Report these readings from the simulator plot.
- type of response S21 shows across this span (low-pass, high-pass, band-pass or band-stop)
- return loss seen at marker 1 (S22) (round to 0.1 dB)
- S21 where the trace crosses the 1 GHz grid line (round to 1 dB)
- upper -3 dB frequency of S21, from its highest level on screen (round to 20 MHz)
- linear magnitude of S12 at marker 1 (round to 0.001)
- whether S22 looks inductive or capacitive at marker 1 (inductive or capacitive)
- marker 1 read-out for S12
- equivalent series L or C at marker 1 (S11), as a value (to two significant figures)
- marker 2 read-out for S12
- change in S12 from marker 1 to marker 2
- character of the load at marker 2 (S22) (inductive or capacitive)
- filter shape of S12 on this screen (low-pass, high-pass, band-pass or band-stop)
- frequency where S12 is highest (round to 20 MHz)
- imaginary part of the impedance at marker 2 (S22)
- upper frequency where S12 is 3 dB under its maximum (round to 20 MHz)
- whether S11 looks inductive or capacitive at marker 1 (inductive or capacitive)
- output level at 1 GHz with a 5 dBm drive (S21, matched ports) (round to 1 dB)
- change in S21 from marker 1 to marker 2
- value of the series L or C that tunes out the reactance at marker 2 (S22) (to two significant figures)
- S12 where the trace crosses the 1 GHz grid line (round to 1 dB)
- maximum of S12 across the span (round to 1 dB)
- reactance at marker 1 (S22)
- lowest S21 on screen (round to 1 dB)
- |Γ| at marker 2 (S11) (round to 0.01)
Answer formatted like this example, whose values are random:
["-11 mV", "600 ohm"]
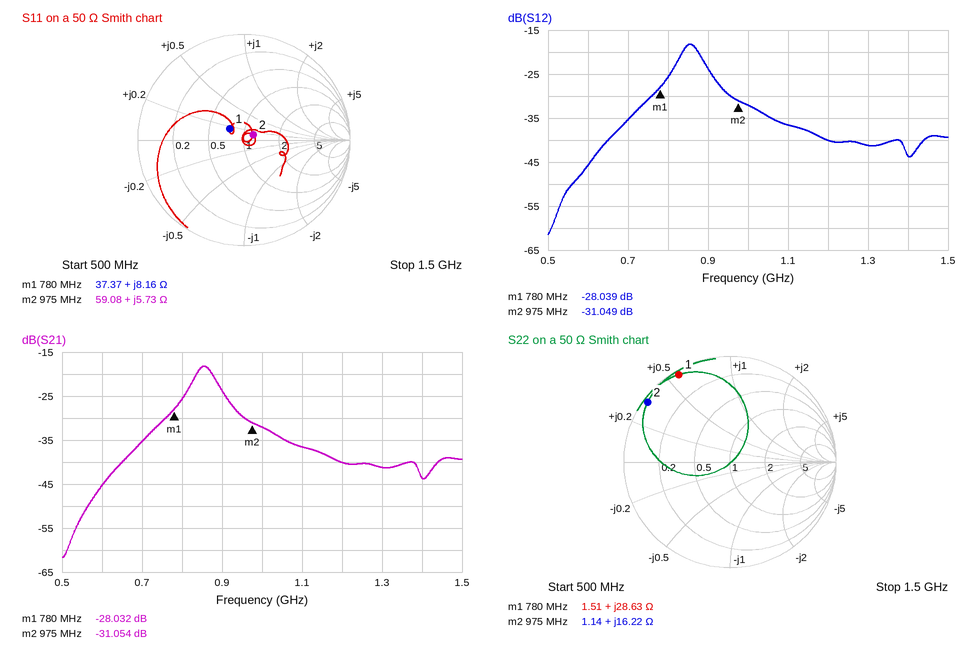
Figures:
["band-pass", "0.4 dB", "-32 dB", "880 MHz", "0.040", "inductive", "-28.039 dB", "1.7 nH", "-31.049 dB", "-3.010 dB", "inductive", "band-pass", "860 MHz", "+16.22 Ω", "880 MHz", "inductive", "-27 dBm", "-3.022 dB", "10 pF", "-32 dB", "-18 dB", "+28.63 Ω", "-62 dB", "0.10"]
